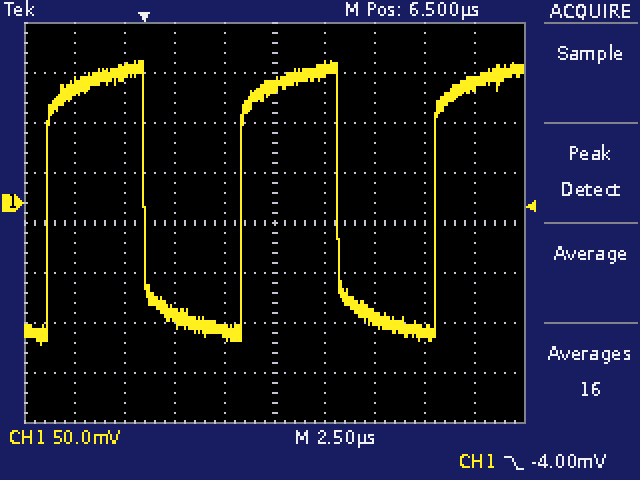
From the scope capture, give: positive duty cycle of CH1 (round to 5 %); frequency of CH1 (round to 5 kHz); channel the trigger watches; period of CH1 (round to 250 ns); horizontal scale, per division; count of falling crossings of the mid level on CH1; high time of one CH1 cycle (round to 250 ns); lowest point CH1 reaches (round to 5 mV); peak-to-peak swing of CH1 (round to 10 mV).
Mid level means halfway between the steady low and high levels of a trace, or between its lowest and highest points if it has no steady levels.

50 %
105 kHz
CH1
9.75 µs
2.5 µs
2
4.75 µs
-140 mV
280 mV
